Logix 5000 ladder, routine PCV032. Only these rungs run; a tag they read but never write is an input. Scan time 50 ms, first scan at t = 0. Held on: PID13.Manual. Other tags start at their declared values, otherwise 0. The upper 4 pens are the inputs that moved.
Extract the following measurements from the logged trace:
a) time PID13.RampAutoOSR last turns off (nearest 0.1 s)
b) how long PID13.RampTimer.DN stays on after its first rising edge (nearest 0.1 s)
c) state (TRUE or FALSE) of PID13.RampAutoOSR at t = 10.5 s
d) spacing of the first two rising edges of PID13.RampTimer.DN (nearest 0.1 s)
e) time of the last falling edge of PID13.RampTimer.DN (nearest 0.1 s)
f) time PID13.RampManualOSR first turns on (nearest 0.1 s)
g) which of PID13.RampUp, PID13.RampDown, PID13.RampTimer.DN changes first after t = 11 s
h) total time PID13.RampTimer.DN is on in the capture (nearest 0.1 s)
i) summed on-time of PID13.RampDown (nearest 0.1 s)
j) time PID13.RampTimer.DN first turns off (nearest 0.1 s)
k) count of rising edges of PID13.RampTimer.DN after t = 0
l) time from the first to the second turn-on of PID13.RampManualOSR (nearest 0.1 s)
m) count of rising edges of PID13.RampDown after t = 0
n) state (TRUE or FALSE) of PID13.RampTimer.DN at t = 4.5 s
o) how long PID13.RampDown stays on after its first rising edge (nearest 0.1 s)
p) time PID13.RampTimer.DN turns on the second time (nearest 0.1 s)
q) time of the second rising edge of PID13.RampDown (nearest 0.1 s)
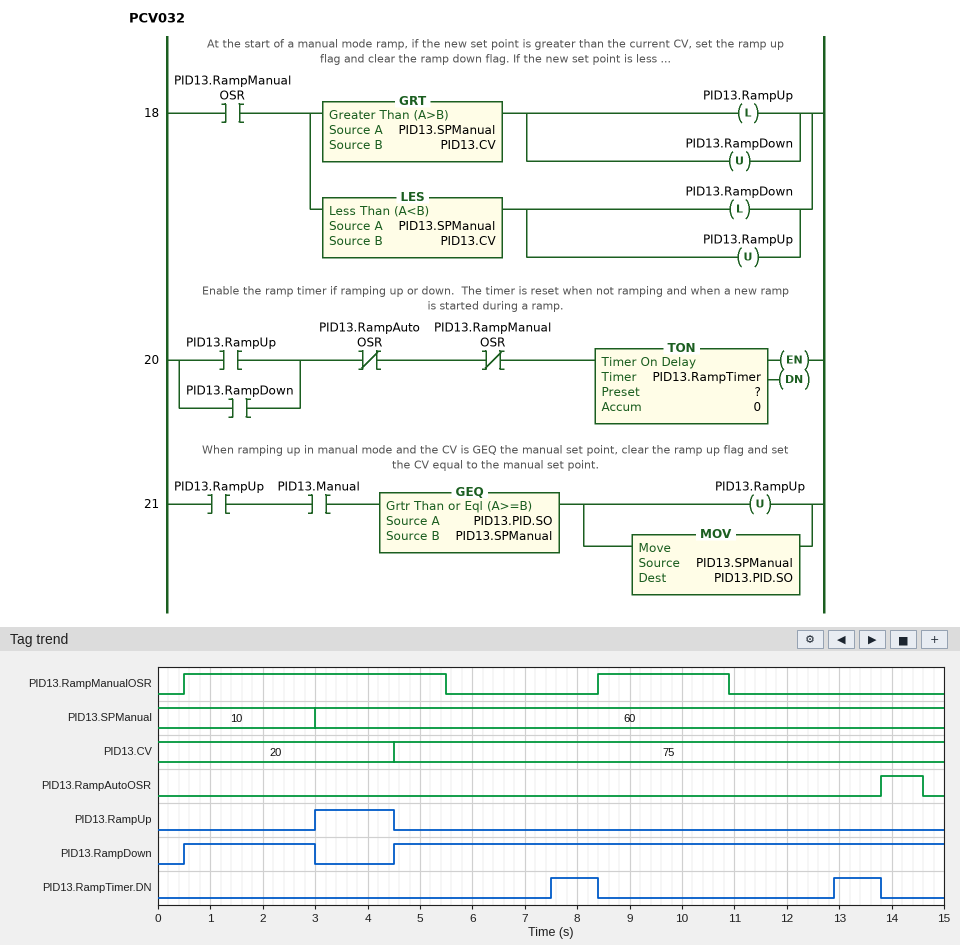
14.6 s
0.9 s
FALSE
5.4 s
13.8 s
0.5 s
PID13.RampTimer.DN
1.8 s
13.0 s
8.4 s
2
7.9 s
2
FALSE
2.5 s
12.9 s
4.5 s
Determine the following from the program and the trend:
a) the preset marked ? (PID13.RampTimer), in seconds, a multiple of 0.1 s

2.0 s
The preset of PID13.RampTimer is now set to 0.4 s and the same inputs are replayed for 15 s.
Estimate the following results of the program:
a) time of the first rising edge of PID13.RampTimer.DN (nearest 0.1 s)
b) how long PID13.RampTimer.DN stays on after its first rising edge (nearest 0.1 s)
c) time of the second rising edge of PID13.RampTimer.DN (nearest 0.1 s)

5.9 s
2.5 s
11.3 s
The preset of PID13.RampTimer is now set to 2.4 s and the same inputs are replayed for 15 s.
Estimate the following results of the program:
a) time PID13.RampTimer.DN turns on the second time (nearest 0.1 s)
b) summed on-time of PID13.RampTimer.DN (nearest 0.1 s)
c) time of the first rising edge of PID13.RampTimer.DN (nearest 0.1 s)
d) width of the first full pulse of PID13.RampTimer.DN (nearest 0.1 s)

13.3 s
1.0 s
7.9 s
0.5 s
